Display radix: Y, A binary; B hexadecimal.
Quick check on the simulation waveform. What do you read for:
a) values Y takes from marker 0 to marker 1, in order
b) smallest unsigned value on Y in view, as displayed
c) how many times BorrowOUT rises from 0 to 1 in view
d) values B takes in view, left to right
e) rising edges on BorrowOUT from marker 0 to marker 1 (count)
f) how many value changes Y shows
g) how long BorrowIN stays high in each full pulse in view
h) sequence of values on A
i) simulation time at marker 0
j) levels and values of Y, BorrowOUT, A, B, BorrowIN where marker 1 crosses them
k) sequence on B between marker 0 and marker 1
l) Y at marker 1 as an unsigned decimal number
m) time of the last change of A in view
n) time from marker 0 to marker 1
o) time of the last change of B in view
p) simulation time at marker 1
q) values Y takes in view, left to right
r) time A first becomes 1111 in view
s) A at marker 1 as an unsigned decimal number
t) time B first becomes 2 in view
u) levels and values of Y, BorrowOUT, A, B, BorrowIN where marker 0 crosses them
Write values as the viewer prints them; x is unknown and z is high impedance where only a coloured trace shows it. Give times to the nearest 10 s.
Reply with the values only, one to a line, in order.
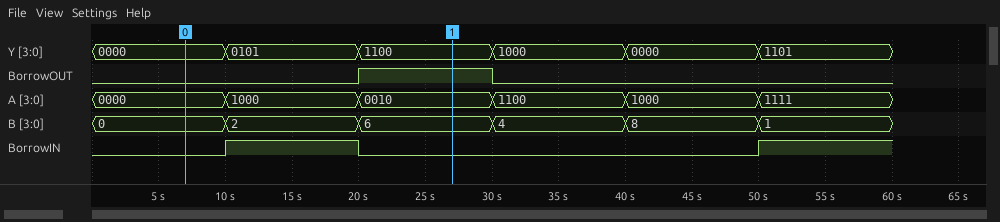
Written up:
0000, 0101, 1100
0000
1
0, 2, 6, 4, 8, 1
1
5
10 s
0000, 1000, 0010, 1100, 1000, 1111
10 s
Y=1100, BorrowOUT=1, A=0010, B=6, BorrowIN=0
0, 2, 6
12
50 s
20 s
50 s
30 s
0000, 0101, 1100, 1000, 0000, 1101
50 s
2
10 s
Y=0000, BorrowOUT=0, A=0000, B=0, BorrowIN=0
